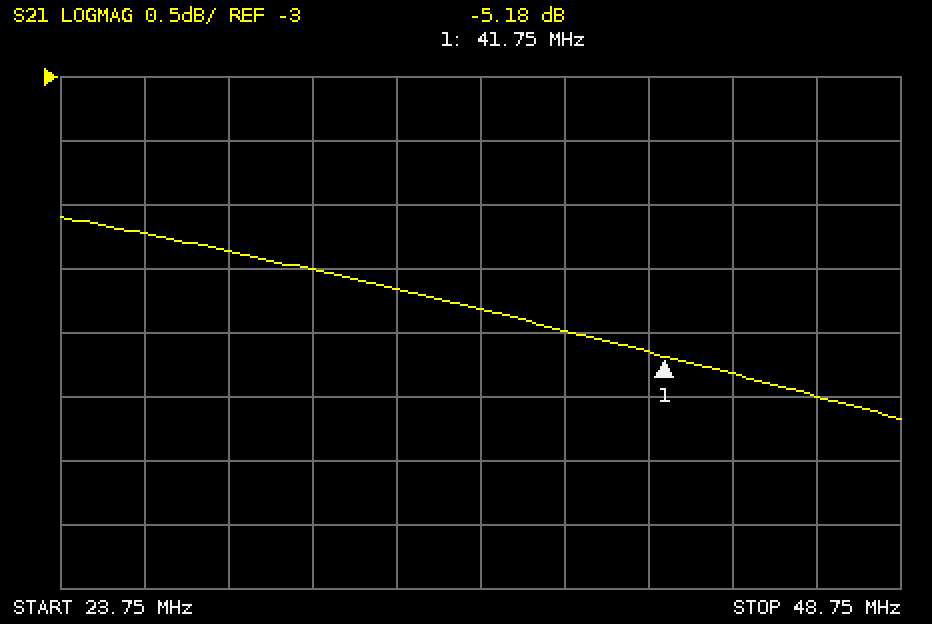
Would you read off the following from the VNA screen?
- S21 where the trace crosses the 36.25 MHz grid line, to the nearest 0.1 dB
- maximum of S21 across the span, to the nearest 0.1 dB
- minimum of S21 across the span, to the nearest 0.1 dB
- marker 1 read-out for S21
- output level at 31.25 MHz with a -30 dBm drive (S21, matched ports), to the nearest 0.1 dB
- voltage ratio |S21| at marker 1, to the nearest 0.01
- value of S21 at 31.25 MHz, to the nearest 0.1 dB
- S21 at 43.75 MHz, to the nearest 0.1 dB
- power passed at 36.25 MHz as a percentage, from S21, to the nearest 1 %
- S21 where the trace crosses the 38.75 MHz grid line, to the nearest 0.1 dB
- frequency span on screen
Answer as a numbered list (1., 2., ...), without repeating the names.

1. -4.8 dB
2. -4.1 dB
3. -5.7 dB
4. -5.18 dB
5. -34.5 dBm
6. 0.55
7. -4.5 dB
8. -5.3 dB
9. 33 %
10. -5.0 dB
11. 25 MHz
